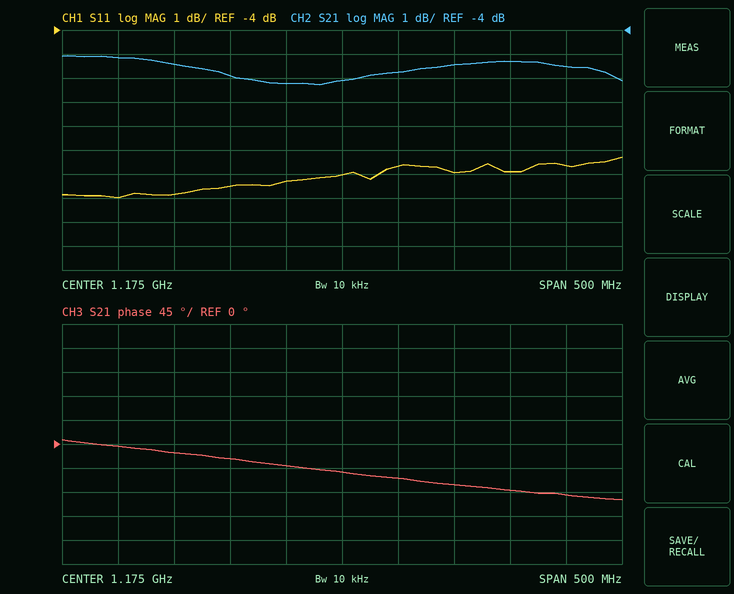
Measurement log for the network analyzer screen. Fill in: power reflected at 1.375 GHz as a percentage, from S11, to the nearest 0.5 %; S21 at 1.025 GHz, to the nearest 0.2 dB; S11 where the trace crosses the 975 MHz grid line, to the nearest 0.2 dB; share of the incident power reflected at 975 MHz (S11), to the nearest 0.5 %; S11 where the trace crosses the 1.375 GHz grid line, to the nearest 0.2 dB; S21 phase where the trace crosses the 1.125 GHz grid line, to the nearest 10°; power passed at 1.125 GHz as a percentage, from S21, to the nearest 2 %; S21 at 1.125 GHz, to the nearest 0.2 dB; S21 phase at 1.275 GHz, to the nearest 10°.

11.0 %
-5.4 dB
-11.0 dB
8.0 %
-9.6 dB
-40°
24 %
-6.2 dB
-80°
